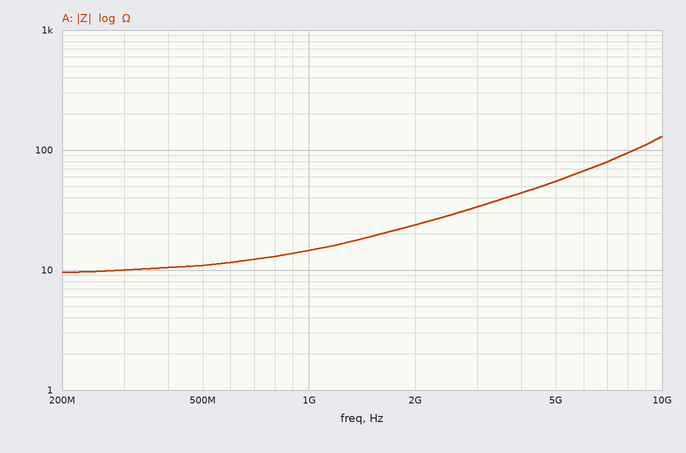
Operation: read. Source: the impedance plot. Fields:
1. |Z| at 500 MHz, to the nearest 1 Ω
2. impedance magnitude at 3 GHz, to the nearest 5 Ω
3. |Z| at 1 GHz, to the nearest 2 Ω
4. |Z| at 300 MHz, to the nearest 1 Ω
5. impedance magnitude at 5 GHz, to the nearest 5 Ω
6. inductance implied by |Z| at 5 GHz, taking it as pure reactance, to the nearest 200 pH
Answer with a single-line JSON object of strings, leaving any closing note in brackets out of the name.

{"|Z| at 500 MHz, to the nearest 1 Ω": "11 Ω", "impedance magnitude at 3 GHz, to the nearest 5 Ω": "35 Ω", "|Z| at 1 GHz, to the nearest 2 Ω": "14 Ω", "|Z| at 300 MHz, to the nearest 1 Ω": "10 Ω", "impedance magnitude at 5 GHz, to the nearest 5 Ω": "55 Ω", "inductance implied by |Z| at 5 GHz, taking it as pure reactance, to the nearest 200 pH": "1.8 nH"}
